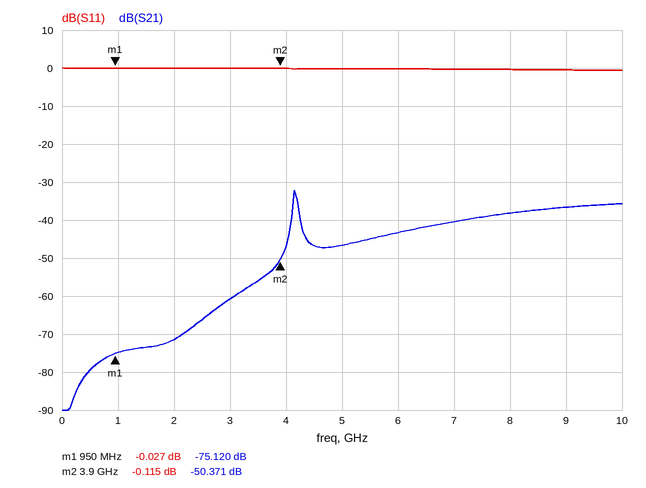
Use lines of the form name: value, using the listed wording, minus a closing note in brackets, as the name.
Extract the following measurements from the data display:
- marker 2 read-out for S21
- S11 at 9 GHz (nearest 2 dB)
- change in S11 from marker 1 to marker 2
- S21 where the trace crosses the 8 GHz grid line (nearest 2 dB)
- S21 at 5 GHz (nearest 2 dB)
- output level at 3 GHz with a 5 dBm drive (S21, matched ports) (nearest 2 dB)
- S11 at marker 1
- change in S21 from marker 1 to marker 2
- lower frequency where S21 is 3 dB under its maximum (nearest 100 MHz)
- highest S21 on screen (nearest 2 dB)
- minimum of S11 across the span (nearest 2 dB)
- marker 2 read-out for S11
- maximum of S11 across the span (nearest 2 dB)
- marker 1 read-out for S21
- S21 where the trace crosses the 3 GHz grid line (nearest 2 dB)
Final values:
marker 2 read-out for S21: -50.371 dB
S11 at 9 GHz: 0 dB
change in S11 from marker 1 to marker 2: -0.088 dB
S21 where the trace crosses the 8 GHz grid line: -38 dB
S21 at 5 GHz: -46 dB
output level at 3 GHz with a 5 dBm drive (S21, matched ports): -56 dBm
S11 at marker 1: -0.027 dB
change in S21 from marker 1 to marker 2: 24.749 dB
lower frequency where S21 is 3 dB under its maximum: 4.1 GHz
highest S21 on screen: -32 dB
minimum of S11 across the span: 0 dB
marker 2 read-out for S11: -0.115 dB
maximum of S11 across the span: 0 dB
marker 1 read-out for S21: -75.120 dB
S21 where the trace crosses the 3 GHz grid line: -60 dB
